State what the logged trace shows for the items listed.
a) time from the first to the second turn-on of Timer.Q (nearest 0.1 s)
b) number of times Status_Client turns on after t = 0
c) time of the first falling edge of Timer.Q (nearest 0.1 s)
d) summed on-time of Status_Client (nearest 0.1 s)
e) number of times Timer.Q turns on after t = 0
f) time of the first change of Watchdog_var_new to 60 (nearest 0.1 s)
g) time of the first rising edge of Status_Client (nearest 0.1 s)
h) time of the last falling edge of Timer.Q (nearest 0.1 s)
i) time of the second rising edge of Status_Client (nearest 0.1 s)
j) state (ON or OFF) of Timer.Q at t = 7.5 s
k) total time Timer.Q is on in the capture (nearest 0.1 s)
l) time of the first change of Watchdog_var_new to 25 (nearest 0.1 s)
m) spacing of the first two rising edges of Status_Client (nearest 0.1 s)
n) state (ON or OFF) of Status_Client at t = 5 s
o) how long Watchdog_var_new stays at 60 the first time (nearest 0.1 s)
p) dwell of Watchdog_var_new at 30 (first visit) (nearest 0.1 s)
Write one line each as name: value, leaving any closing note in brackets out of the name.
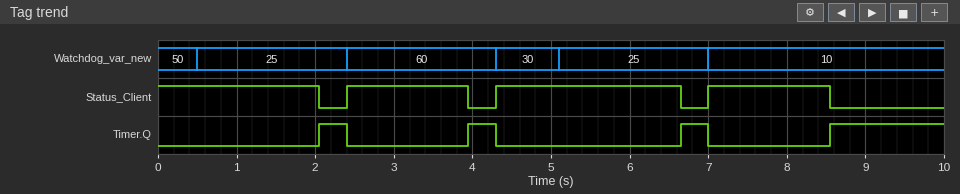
time from the first to the second turn-on of Timer.Q: 1.9 s
number of times Status_Client turns on after t = 0: 3
time of the first falling edge of Timer.Q: 2.4 s
summed on-time of Status_Client: 7.5 s
number of times Timer.Q turns on after t = 0: 4
time of the first change of Watchdog_var_new to 60: 2.4 s
time of the first rising edge of Status_Client: 2.4 s
time of the last falling edge of Timer.Q: 7.0 s
time of the second rising edge of Status_Client: 4.3 s
state (ON or OFF) of Timer.Q at t = 7.5 s: OFF
total time Timer.Q is on in the capture: 2.5 s
time of the first change of Watchdog_var_new to 25: 0.5 s
spacing of the first two rising edges of Status_Client: 1.9 s
state (ON or OFF) of Status_Client at t = 5 s: ON
how long Watchdog_var_new stays at 60 the first time: 1.9 s
dwell of Watchdog_var_new at 30 (first visit): 0.8 s
